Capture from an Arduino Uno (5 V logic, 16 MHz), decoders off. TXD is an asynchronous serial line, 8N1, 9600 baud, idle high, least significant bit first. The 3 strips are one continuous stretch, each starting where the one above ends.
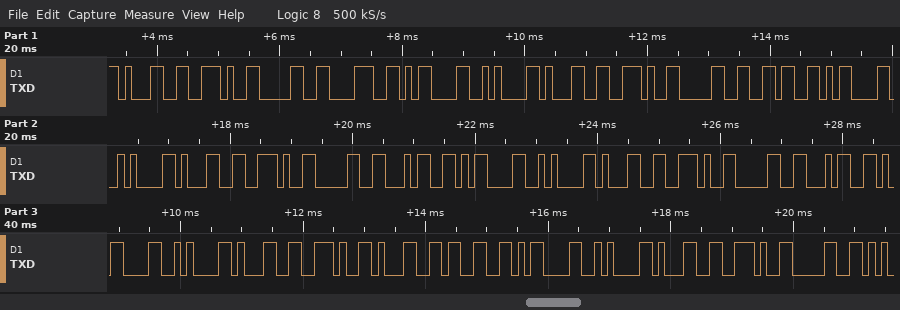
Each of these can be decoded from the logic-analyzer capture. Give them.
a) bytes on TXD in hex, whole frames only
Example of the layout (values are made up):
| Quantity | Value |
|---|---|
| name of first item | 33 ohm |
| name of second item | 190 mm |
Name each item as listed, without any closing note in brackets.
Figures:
| Quantity | Value |
|---|---|
| bytes on TXD in hex, whole frames only | 31 2E 30 38 0D 0A 31 2E 30 36 0D 0A 31 2E 30 34 0D 0A 31 2E 30 34 0D 0A 31 2E 31 33 0D 0A 31 2E 30 |
